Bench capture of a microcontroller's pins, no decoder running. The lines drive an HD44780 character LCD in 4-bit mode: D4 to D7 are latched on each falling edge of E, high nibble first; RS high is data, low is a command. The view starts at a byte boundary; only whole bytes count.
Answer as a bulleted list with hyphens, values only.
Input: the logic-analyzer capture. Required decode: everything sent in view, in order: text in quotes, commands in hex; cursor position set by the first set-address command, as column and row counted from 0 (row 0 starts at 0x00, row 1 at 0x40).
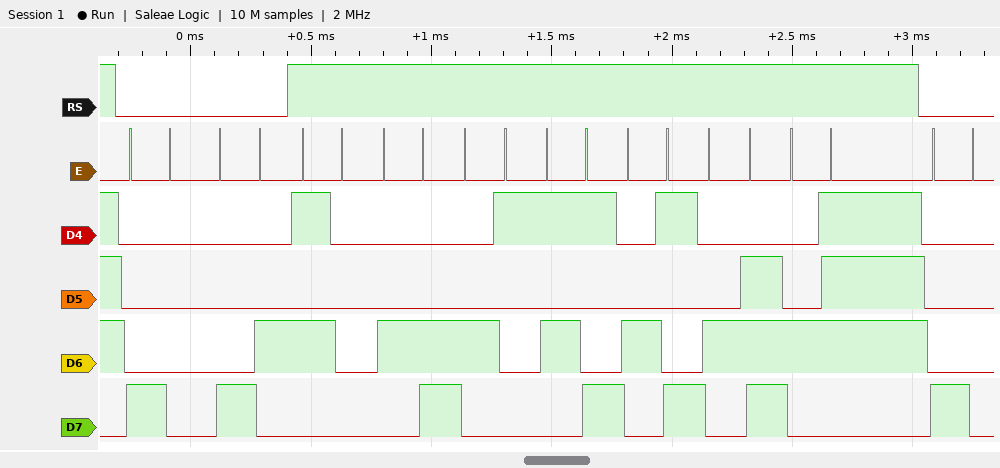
- 0x80 0x84 "PLAYING" 0x80
- column 0, row 0
